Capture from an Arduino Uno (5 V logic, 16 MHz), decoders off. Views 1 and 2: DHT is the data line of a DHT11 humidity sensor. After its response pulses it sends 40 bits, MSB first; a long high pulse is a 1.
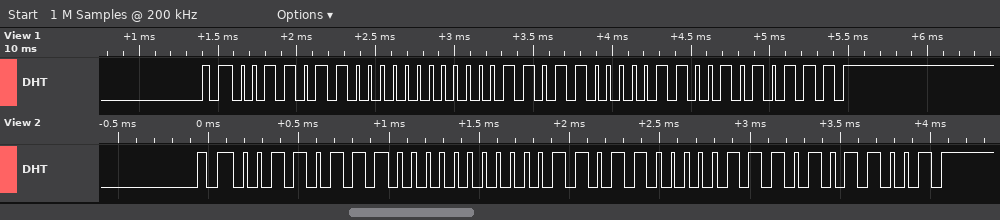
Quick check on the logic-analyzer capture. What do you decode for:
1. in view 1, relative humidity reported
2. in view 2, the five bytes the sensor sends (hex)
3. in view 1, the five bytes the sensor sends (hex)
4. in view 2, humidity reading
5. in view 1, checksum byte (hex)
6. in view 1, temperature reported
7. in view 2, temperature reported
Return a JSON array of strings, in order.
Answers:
["54 %", "37 00 1B 07 59", "36 00 1B 06 57", "55 %", "0x57", "27.6 °C", "27.7 °C"]
